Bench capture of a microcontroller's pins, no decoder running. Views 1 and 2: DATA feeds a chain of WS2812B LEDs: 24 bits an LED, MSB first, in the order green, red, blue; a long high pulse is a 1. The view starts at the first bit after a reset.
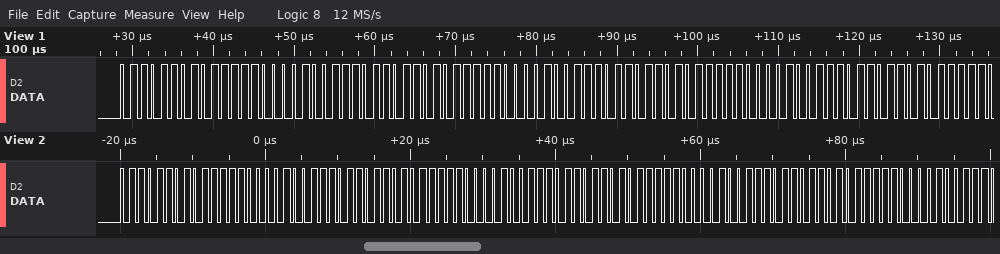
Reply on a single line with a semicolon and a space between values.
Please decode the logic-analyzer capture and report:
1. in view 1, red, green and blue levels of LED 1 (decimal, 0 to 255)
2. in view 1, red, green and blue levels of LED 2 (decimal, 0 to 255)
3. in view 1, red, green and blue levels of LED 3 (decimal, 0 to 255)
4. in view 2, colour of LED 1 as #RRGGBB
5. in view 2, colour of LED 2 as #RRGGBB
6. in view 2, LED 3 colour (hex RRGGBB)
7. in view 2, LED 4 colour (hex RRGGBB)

124, 109, 39; 124, 109, 39; 124, 109, 39; #7C6D27; #7C6D27; #7C6D27; #7C6D27
